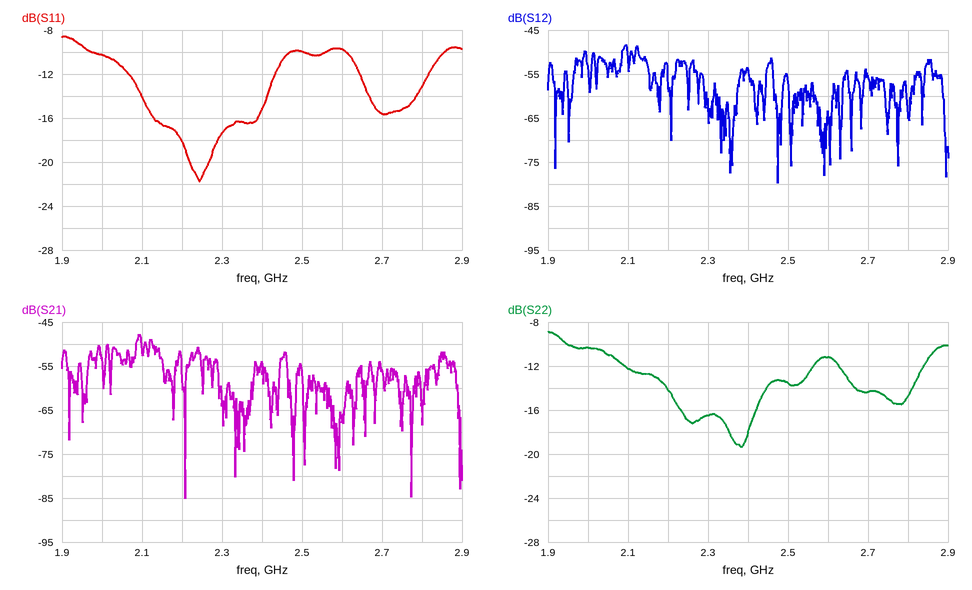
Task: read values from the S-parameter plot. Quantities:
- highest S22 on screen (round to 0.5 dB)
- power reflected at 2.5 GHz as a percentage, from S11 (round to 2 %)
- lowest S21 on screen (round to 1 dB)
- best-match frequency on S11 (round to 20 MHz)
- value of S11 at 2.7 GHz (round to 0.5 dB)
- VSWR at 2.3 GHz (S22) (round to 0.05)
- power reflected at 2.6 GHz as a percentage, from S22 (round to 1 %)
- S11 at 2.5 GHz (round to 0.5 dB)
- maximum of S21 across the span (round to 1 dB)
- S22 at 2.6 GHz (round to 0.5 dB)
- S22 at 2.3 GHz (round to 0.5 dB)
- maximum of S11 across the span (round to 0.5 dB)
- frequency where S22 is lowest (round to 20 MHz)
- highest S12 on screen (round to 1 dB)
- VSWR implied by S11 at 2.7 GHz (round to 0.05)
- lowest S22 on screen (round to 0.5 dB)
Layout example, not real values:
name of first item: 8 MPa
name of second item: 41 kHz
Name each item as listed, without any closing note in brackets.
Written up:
highest S22 on screen: -9.0 dB
power reflected at 2.5 GHz as a percentage, from S11: 10 %
lowest S21 on screen: -85 dB
best-match frequency on S11: 2.24 GHz
value of S11 at 2.7 GHz: -15.5 dB
VSWR at 2.3 GHz (S22): 1.35
power reflected at 2.6 GHz as a percentage, from S22: 8 %
S11 at 2.5 GHz: -10.0 dB
maximum of S21 across the span: -48 dB
S22 at 2.6 GHz: -11.0 dB
S22 at 2.3 GHz: -16.5 dB
maximum of S11 across the span: -8.5 dB
frequency where S22 is lowest: 2.38 GHz
highest S12 on screen: -48 dB
VSWR implied by S11 at 2.7 GHz: 1.40
lowest S22 on screen: -19.5 dB
